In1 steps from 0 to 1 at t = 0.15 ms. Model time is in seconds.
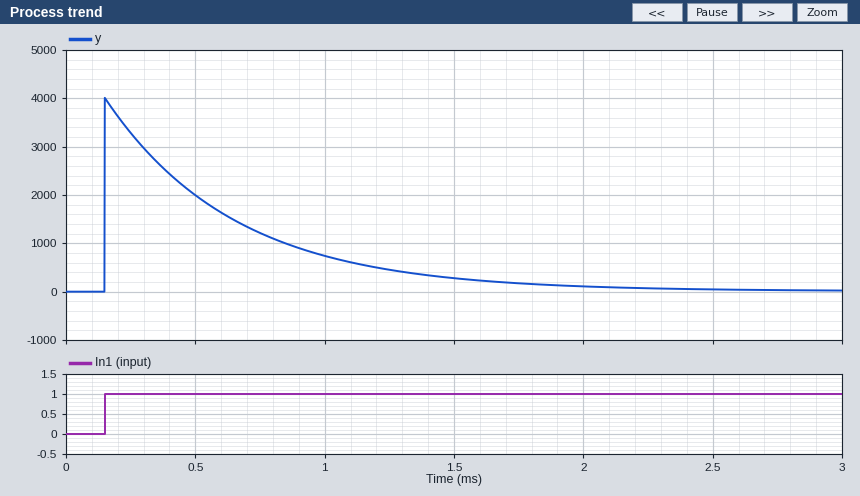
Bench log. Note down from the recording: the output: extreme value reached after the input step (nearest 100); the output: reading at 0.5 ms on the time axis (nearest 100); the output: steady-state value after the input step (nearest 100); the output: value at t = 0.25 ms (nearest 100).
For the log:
4000
2000
0
3300
